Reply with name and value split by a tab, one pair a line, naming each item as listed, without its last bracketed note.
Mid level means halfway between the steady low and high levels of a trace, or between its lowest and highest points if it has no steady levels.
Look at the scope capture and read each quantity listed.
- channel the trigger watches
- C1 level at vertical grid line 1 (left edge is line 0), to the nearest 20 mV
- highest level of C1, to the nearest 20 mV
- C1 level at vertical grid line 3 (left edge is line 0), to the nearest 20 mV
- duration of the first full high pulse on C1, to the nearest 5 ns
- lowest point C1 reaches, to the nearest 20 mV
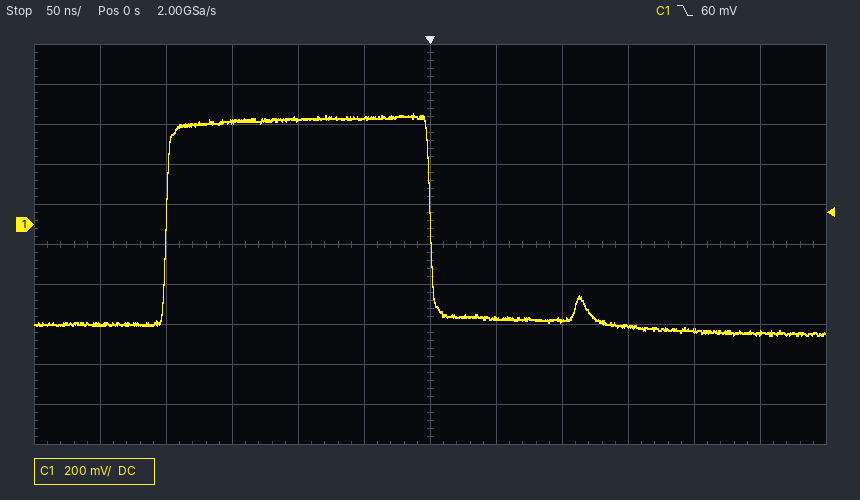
channel the trigger watches	C1
C1 level at vertical grid line 1 (left edge is line 0), to the nearest 20 mV	-500 mV
highest level of C1, to the nearest 20 mV	560 mV
C1 level at vertical grid line 3 (left edge is line 0), to the nearest 20 mV	520 mV
duration of the first full high pulse on C1, to the nearest 5 ns	200 ns
lowest point C1 reaches, to the nearest 20 mV	-560 mV
